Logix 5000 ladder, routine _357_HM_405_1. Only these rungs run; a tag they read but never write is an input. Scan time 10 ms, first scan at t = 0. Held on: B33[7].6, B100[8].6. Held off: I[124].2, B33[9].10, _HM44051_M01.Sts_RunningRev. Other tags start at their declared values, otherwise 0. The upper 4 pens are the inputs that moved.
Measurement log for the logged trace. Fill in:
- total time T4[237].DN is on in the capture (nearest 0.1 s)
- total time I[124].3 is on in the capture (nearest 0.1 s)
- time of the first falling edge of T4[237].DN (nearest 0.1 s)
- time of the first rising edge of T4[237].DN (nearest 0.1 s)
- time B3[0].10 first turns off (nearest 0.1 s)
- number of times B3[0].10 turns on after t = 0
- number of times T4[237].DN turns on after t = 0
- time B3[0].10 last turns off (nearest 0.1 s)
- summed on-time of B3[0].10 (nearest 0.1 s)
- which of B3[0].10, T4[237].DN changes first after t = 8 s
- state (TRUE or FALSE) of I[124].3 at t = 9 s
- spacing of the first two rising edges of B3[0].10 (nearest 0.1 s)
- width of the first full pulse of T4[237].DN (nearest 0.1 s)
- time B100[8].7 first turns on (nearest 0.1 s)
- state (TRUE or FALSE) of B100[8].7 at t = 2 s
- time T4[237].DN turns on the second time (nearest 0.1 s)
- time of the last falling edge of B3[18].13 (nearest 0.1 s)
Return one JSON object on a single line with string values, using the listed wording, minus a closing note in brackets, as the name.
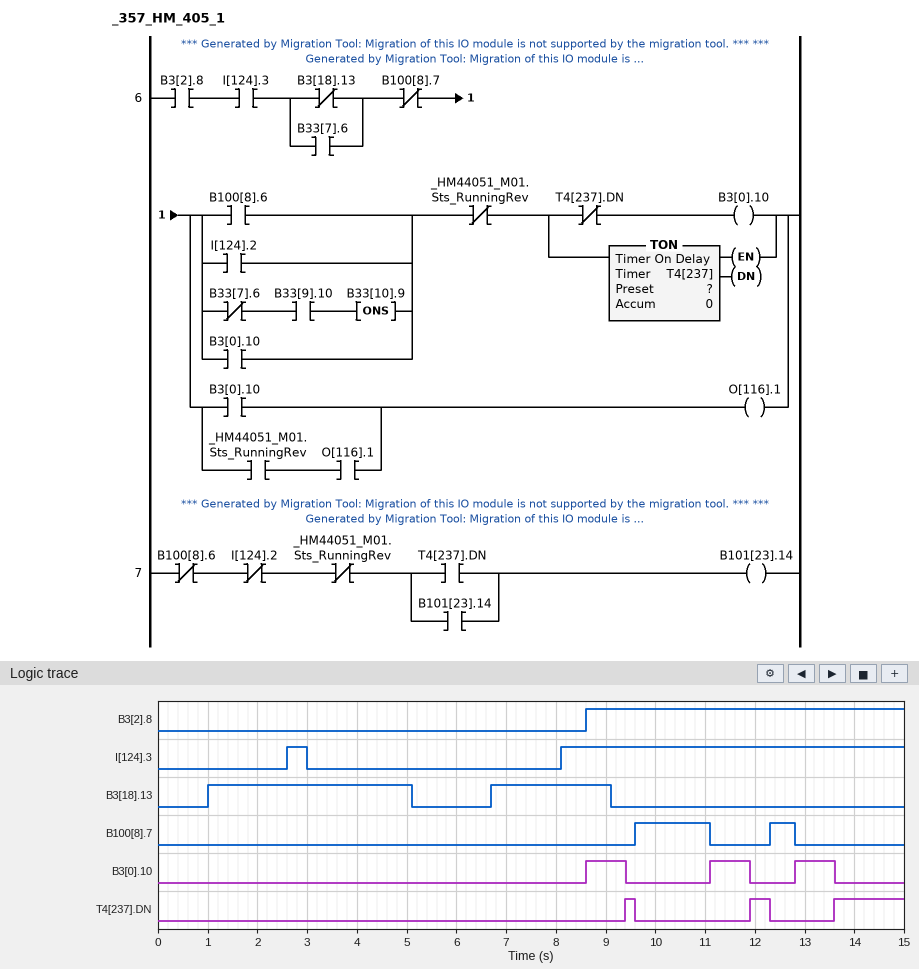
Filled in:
{"total time T4[237].DN is on in the capture": "2.0 s", "total time I[124].3 is on in the capture": "7.3 s", "time of the first falling edge of T4[237].DN": "9.6 s", "time of the first rising edge of T4[237].DN": "9.4 s", "time B3[0].10 first turns off": "9.4 s", "number of times B3[0].10 turns on after t = 0": "3", "number of times T4[237].DN turns on after t = 0": "3", "time B3[0].10 last turns off": "13.6 s", "summed on-time of B3[0].10": "2.4 s", "which of B3[0].10, T4[237].DN changes first after t = 8 s": "B3[0].10", "state (TRUE or FALSE) of I[124].3 at t = 9 s": "TRUE", "spacing of the first two rising edges of B3[0].10": "2.5 s", "width of the first full pulse of T4[237].DN": "0.2 s", "time B100[8].7 first turns on": "9.6 s", "state (TRUE or FALSE) of B100[8].7 at t = 2 s": "FALSE", "time T4[237].DN turns on the second time": "11.9 s", "time of the last falling edge of B3[18].13": "9.1 s"}
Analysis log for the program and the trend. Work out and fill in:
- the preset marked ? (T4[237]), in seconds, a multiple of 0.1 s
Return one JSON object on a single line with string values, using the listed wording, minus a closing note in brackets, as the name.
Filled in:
{"the preset marked ? (T4[237]), in seconds, a multiple of 0.1 s": "0.8 s"}
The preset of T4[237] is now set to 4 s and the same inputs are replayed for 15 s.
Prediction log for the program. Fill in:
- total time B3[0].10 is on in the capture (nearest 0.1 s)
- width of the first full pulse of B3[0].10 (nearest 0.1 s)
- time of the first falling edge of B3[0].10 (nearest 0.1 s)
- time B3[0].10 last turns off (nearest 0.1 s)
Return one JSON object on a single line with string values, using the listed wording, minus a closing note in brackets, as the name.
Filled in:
{"total time B3[0].10 is on in the capture": "4.4 s", "width of the first full pulse of B3[0].10": "1.0 s", "time of the first falling edge of B3[0].10": "9.6 s", "time B3[0].10 last turns off": "12.3 s"}
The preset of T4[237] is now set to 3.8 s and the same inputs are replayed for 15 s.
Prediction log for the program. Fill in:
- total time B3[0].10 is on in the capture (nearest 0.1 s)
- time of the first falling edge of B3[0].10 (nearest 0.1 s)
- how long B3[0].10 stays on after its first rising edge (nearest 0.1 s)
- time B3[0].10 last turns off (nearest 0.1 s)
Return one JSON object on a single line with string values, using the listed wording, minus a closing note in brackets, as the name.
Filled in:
{"total time B3[0].10 is on in the capture": "4.4 s", "time of the first falling edge of B3[0].10": "9.6 s", "how long B3[0].10 stays on after its first rising edge": "1.0 s", "time B3[0].10 last turns off": "12.3 s"}
